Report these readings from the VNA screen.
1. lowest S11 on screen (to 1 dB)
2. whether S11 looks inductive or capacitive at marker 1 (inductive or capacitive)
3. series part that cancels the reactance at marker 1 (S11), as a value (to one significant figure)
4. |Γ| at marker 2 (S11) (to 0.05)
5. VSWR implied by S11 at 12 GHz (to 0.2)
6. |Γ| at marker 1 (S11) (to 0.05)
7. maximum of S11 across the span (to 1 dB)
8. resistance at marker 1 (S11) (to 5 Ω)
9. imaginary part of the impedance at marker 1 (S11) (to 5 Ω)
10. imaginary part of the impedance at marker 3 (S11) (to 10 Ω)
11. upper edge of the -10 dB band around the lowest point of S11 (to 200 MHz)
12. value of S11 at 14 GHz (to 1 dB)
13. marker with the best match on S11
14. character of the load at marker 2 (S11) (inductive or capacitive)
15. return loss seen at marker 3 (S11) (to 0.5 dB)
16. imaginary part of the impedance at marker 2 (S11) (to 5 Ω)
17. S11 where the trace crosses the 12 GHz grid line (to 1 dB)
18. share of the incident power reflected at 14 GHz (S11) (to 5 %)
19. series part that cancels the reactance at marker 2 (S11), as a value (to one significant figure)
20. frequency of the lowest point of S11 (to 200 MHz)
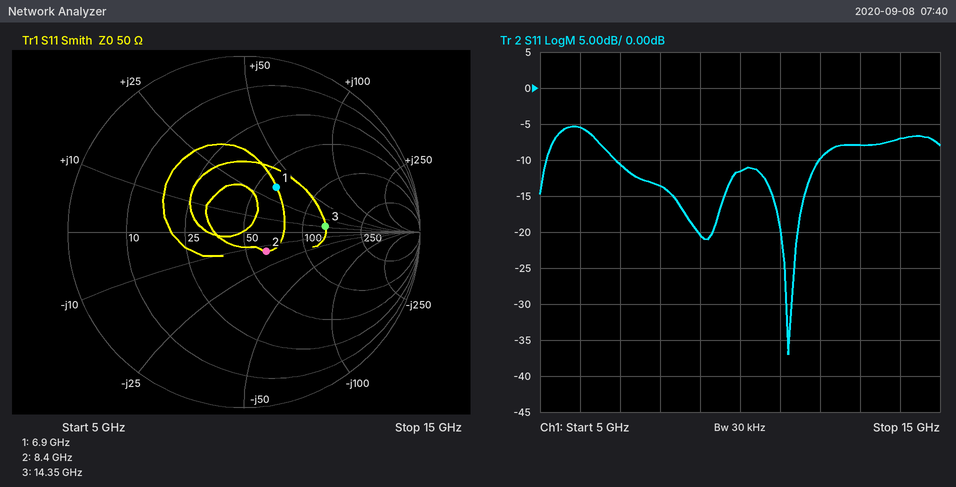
-37 dB
inductive
700 fF
0.15
2.0
0.30
-5 dB
60 Ω
+35 Ω
+10 Ω
12.0 GHz
-7 dB
marker 2
capacitive
6.5 dB
-15 Ω
-10 dB
20 %
300 pH
11.2 GHz
